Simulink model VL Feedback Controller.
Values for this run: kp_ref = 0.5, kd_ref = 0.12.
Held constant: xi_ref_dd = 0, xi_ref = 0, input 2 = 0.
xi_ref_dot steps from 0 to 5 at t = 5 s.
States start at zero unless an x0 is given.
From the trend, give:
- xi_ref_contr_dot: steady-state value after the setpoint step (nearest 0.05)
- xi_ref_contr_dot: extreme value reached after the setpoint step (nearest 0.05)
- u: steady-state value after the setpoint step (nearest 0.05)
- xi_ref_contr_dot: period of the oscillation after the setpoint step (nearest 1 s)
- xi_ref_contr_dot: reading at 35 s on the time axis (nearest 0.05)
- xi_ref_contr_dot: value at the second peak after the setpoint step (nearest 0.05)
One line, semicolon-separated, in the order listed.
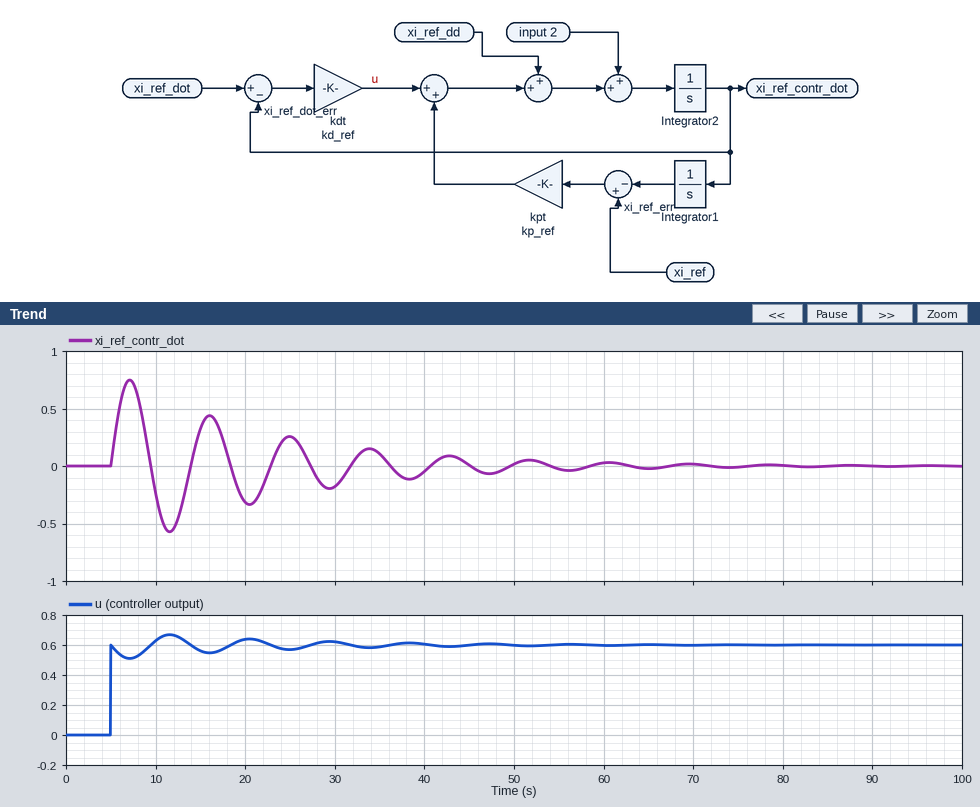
0.00; 0.75; 0.60; 9 s; 0.10; 0.45
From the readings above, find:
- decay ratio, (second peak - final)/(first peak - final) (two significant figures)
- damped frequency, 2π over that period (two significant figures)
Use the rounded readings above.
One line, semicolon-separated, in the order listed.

0.60; 0.70 rad/s
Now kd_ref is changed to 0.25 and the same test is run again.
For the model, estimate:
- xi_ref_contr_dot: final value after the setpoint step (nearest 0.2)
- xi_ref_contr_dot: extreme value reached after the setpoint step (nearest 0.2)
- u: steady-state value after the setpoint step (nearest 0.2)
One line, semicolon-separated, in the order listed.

0.0; 1.4; 1.2
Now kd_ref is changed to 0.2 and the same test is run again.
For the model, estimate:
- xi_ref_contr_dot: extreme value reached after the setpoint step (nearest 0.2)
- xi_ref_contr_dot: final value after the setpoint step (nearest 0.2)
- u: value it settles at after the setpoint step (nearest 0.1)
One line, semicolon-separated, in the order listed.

1.2; 0.0; 1.0
